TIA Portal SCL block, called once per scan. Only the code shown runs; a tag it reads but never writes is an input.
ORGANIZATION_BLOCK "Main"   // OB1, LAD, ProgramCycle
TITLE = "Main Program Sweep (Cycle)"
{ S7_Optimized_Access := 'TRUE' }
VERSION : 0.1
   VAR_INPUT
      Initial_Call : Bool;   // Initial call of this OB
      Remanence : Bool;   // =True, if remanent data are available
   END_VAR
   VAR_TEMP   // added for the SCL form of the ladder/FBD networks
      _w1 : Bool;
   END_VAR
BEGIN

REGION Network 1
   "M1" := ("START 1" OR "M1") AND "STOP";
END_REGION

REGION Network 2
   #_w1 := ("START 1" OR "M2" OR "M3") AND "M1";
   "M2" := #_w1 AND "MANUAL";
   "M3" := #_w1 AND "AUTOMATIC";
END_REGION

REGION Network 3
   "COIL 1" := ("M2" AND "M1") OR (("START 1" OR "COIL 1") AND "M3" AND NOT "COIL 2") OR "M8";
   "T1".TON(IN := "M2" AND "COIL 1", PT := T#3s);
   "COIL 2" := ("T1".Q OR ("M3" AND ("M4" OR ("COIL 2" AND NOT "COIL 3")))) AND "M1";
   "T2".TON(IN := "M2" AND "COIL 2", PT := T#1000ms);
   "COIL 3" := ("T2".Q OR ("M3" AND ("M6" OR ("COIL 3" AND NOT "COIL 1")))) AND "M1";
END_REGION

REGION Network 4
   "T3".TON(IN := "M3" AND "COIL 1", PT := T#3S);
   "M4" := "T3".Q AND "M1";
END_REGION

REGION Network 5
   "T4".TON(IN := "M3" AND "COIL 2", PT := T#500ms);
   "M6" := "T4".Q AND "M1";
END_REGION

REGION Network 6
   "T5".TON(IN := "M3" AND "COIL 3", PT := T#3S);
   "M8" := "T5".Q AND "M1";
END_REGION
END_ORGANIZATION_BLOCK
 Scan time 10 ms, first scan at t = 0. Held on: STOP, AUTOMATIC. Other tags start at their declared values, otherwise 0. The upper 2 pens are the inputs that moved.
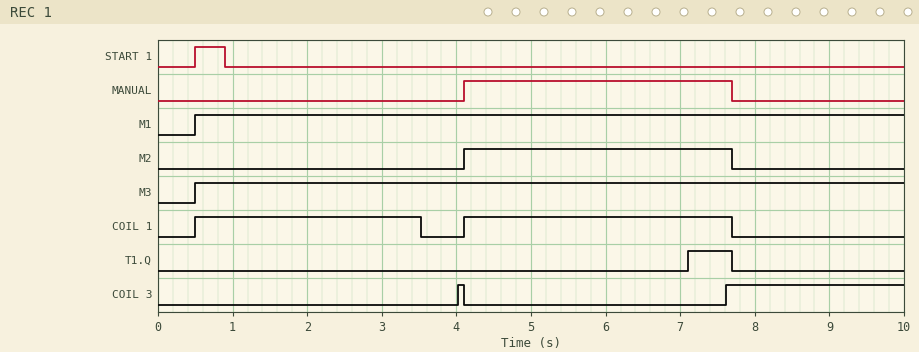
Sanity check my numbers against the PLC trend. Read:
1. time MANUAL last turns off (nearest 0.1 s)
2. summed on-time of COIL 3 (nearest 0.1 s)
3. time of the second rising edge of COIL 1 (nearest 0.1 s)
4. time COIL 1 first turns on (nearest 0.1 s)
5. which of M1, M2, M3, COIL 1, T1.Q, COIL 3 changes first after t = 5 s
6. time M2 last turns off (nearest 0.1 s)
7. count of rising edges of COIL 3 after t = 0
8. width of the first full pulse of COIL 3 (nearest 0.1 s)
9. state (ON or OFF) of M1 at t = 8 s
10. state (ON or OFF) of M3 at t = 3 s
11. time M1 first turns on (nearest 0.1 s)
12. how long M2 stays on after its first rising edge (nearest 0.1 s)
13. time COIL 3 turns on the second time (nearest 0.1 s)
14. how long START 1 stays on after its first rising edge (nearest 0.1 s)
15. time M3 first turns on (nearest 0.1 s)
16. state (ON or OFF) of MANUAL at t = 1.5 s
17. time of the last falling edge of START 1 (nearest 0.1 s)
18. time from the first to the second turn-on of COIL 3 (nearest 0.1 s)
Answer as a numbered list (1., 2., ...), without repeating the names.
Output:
1. 7.7 s
2. 2.5 s
3. 4.1 s
4. 0.5 s
5. T1.Q
6. 7.7 s
7. 2
8. 0.1 s
9. ON
10. ON
11. 0.5 s
12. 3.6 s
13. 7.6 s
14. 0.4 s
15. 0.5 s
16. OFF
17. 0.9 s
18. 3.6 s
